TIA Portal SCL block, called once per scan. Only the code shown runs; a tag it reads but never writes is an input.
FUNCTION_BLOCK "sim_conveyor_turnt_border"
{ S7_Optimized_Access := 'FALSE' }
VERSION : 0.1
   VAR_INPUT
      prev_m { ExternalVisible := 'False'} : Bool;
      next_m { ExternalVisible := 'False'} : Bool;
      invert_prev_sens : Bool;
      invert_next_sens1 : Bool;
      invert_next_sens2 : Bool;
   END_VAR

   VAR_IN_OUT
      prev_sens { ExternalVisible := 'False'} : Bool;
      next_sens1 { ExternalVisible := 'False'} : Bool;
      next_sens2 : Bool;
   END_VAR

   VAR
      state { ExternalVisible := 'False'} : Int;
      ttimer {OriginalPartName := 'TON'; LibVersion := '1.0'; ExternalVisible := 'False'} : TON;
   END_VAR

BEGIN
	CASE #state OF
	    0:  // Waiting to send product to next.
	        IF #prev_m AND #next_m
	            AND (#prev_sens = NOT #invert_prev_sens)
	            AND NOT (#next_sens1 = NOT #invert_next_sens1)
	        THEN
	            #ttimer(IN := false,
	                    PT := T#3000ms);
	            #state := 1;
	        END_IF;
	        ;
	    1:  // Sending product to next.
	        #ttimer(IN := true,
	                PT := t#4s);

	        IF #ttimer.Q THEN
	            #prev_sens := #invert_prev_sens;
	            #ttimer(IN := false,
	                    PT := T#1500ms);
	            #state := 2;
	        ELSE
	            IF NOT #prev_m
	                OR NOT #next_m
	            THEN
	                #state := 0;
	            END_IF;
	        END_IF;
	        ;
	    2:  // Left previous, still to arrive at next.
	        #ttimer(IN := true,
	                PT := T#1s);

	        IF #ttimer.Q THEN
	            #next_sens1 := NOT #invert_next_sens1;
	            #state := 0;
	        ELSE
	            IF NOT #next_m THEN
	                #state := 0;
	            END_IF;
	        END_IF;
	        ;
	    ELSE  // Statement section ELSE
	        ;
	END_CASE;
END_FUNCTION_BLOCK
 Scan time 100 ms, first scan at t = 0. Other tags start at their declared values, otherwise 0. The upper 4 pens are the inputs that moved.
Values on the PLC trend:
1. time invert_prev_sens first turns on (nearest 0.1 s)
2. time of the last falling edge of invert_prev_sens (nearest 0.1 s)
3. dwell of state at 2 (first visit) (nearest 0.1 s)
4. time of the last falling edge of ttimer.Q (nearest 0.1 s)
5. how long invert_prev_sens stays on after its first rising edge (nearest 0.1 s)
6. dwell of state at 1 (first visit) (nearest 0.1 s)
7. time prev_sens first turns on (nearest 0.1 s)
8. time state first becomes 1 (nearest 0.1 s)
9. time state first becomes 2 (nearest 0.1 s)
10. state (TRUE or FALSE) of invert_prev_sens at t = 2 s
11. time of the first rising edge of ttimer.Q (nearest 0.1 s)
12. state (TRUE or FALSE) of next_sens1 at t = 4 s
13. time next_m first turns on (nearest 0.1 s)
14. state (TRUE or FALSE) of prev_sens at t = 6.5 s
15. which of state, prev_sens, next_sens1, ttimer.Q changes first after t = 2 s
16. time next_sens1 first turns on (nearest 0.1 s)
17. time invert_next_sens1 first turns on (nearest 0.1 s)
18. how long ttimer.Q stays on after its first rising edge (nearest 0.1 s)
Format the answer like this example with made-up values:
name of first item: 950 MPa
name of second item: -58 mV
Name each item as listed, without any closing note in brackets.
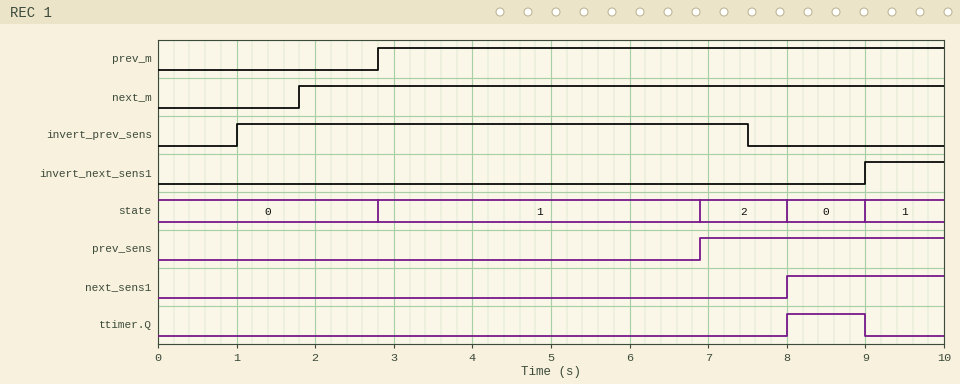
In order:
time invert_prev_sens first turns on: 1.0 s
time of the last falling edge of invert_prev_sens: 7.5 s
dwell of state at 2 (first visit): 1.1 s
time of the last falling edge of ttimer.Q: 9.0 s
how long invert_prev_sens stays on after its first rising edge: 6.5 s
dwell of state at 1 (first visit): 4.1 s
time prev_sens first turns on: 6.9 s
time state first becomes 1: 2.8 s
time state first becomes 2: 6.9 s
state (TRUE or FALSE) of invert_prev_sens at t = 2 s: TRUE
time of the first rising edge of ttimer.Q: 8.0 s
state (TRUE or FALSE) of next_sens1 at t = 4 s: FALSE
time next_m first turns on: 1.8 s
state (TRUE or FALSE) of prev_sens at t = 6.5 s: FALSE
which of state, prev_sens, next_sens1, ttimer.Q changes first after t = 2 s: state
time next_sens1 first turns on: 8.0 s
time invert_next_sens1 first turns on: 9.0 s
how long ttimer.Q stays on after its first rising edge: 1.0 s
